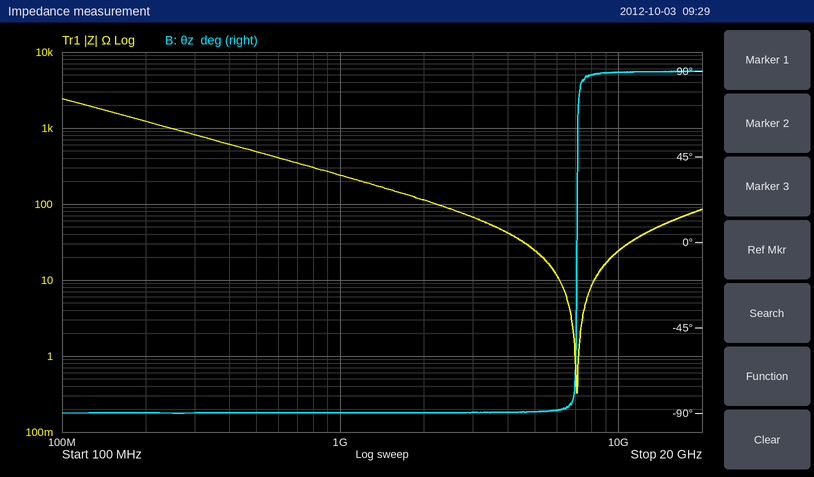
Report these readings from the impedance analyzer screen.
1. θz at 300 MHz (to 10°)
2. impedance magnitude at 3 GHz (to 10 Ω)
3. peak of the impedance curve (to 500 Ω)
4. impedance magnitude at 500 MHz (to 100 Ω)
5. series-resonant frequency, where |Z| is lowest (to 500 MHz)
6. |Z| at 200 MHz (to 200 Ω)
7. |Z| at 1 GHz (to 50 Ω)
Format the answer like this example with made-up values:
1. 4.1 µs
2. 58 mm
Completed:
1. -90°
2. 70 Ω
3. 2.5 kΩ
4. 500 Ω
5. 7.0 GHz
6. 1.2 kΩ
7. 250 Ω
